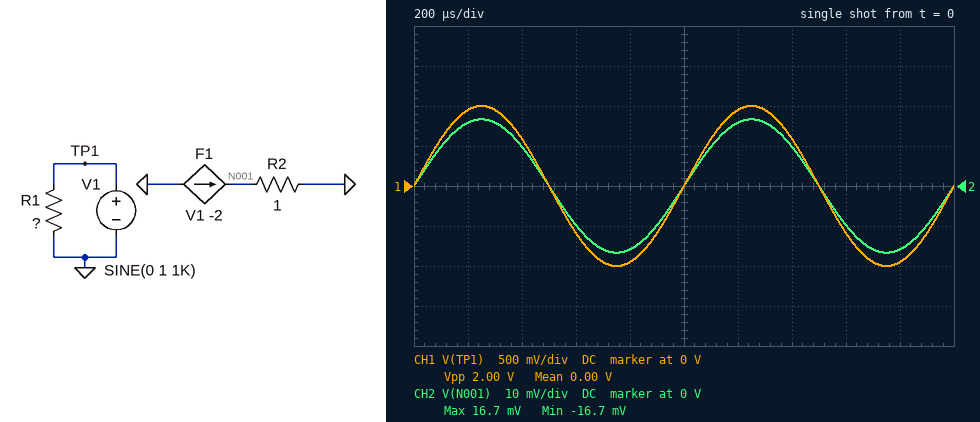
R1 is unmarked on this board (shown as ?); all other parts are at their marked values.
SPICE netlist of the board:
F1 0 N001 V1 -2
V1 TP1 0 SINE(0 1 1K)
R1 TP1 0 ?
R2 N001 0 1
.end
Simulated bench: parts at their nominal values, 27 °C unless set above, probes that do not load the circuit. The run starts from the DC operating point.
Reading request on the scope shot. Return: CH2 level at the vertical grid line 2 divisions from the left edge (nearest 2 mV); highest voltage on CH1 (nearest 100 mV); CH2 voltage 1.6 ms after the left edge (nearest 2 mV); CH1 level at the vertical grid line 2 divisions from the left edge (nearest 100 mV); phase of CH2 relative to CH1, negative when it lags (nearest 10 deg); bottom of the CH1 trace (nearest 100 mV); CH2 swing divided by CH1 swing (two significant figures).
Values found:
10 mV
1.0 V
-10 mV
600 mV
0 deg
-1.0 V
0.017
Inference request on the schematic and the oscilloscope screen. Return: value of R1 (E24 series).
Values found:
120 Ω
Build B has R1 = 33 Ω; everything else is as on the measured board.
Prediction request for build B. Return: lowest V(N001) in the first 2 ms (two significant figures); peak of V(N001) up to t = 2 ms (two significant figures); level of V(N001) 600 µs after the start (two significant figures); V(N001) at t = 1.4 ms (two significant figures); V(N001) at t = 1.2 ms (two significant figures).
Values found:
-61 mV
61 mV
-36 mV
36 mV
58 mV
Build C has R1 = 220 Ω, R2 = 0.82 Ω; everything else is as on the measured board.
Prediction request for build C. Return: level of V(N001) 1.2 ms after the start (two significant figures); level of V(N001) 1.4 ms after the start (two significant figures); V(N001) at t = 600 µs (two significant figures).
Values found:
7.1 mV
4.4 mV
-4.4 mV
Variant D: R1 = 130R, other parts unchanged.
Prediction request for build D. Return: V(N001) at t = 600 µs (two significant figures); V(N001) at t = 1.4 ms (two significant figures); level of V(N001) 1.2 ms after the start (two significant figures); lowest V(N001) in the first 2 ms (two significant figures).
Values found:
-9.0 mV
9.0 mV
15 mV
-15 mV
